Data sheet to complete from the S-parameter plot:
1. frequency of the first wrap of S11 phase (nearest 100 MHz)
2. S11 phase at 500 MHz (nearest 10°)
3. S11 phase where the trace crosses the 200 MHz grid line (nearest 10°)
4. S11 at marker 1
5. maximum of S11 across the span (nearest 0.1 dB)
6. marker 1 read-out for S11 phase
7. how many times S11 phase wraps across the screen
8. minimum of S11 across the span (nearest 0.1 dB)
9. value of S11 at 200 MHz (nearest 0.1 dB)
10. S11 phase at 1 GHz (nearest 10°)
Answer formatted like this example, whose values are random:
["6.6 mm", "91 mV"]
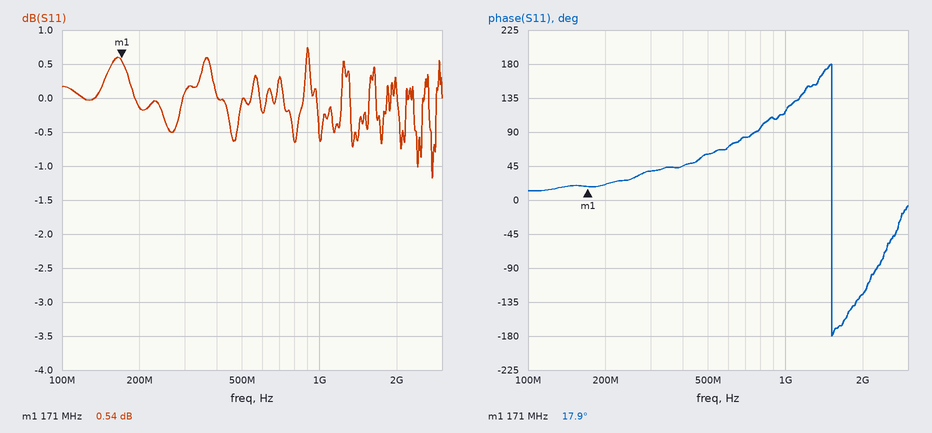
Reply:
["1.5 GHz", "60°", "20°", "0.54 dB", "0.7 dB", "17.9°", "1", "-1.2 dB", "-0.1 dB", "120°"]
